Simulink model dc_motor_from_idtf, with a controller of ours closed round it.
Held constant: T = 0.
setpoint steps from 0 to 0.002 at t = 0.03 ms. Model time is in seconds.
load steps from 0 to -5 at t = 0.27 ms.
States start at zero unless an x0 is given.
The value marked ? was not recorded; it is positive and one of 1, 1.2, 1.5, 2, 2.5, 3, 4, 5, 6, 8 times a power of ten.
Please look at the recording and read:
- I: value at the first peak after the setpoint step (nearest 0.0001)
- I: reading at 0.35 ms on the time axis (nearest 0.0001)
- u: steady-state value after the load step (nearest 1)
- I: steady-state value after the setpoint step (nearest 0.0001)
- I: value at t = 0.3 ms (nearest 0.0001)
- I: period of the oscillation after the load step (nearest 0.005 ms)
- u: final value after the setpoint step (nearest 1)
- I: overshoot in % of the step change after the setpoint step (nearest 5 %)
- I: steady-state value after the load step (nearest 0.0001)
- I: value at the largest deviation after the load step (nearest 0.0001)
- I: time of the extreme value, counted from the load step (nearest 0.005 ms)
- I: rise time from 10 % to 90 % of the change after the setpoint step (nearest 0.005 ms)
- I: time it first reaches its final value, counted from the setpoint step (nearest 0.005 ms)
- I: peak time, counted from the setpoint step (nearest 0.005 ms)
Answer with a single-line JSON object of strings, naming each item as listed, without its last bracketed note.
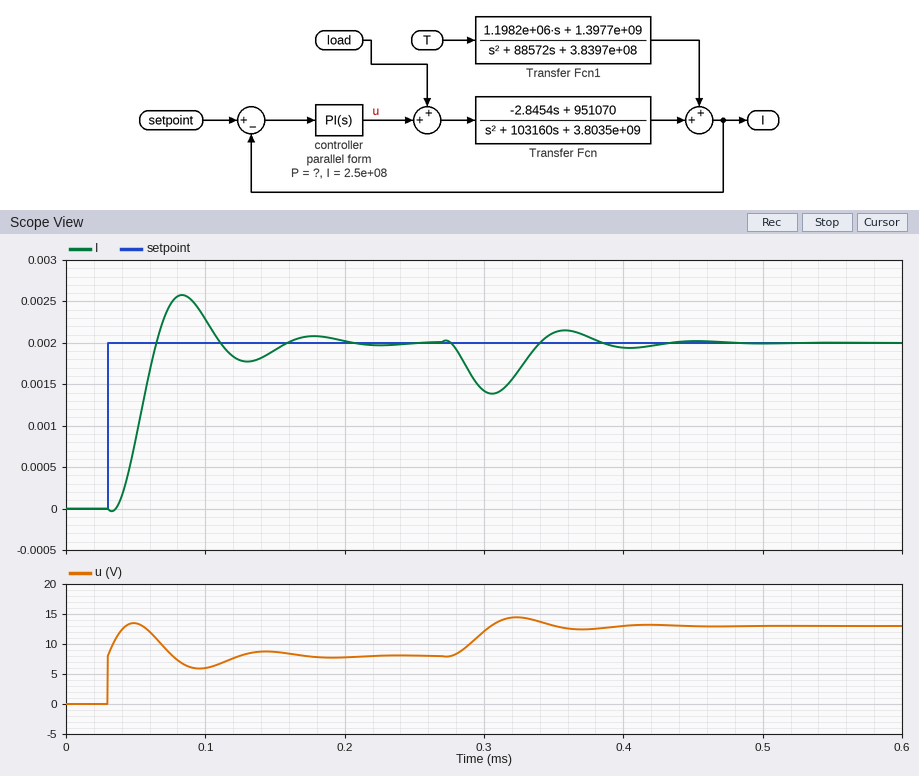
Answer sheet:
{"I: value at the first peak after the setpoint step": "0.0026", "I: reading at 0.35 ms on the time axis": "0.0021", "u: steady-state value after the load step": "13", "I: steady-state value after the setpoint step": "0.0020", "I: value at t = 0.3 ms": "0.0014", "I: period of the oscillation after the load step": "0.100 ms", "u: final value after the setpoint step": "8", "I: overshoot in % of the step change after the setpoint step": "30 %", "I: steady-state value after the load step": "0.0020", "I: value at the largest deviation after the load step": "0.0014", "I: time of the extreme value, counted from the load step": "0.035 ms", "I: rise time from 10 % to 90 % of the change after the setpoint step": "0.020 ms", "I: time it first reaches its final value, counted from the setpoint step": "0.035 ms", "I: peak time, counted from the setpoint step": "0.055 ms"}
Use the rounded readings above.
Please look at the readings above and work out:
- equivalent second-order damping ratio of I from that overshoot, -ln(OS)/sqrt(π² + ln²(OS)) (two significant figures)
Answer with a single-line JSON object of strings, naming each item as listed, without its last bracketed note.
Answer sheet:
{"equivalent second-order damping ratio of I from that overshoot, -ln(OS)/sqrt(π² + ln²(OS))": "0.36"}
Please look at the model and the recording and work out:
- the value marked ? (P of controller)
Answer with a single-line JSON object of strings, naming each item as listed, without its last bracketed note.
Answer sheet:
{"the value marked ?": "4000"}
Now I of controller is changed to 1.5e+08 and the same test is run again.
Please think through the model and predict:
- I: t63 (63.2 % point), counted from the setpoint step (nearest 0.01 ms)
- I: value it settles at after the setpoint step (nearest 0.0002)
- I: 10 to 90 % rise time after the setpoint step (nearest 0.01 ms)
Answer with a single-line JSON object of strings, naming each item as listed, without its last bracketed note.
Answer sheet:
{"I: t63 (63.2 % point), counted from the setpoint step": "0.03 ms", "I: value it settles at after the setpoint step": "0.0020", "I: 10 to 90 % rise time after the setpoint step": "0.03 ms"}
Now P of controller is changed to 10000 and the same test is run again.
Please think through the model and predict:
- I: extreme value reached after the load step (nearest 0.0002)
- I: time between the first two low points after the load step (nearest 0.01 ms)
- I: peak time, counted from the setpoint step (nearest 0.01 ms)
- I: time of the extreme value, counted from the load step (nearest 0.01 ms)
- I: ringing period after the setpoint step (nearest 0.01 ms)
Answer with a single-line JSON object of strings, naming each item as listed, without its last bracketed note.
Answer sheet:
{"I: extreme value reached after the load step": "0.0016", "I: time between the first two low points after the load step": "0.06 ms", "I: peak time, counted from the setpoint step": "0.03 ms", "I: time of the extreme value, counted from the load step": "0.03 ms", "I: ringing period after the setpoint step": "0.06 ms"}
